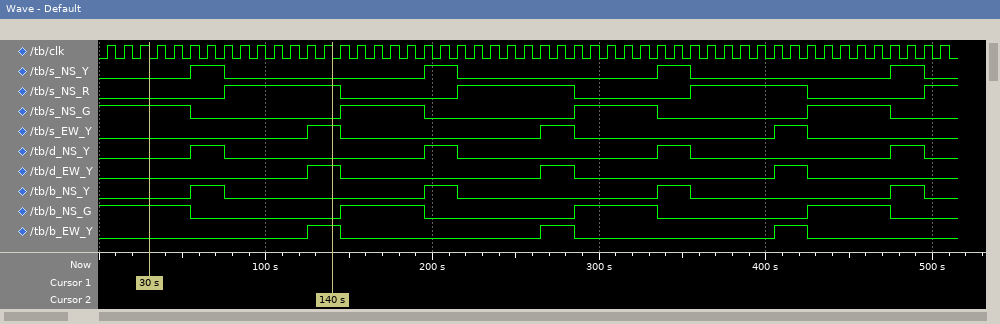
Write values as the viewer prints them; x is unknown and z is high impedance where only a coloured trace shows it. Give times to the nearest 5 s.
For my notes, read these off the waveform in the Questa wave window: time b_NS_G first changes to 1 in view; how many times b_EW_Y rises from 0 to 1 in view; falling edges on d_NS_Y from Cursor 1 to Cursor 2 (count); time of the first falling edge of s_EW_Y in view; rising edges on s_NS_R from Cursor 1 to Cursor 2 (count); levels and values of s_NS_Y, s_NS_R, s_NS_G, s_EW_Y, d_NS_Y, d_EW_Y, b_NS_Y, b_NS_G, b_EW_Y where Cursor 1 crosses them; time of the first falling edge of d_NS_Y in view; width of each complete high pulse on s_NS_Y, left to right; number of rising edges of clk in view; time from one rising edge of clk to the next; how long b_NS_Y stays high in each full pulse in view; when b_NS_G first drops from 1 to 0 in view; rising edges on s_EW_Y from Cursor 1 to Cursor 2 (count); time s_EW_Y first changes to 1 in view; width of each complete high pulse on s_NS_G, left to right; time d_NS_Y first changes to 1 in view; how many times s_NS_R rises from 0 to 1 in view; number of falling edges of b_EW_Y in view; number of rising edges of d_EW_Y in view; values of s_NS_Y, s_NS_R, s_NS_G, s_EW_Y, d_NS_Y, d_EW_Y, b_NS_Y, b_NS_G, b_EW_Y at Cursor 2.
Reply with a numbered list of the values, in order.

1. 145 s
2. 3
3. 1
4. 145 s
5. 1
6. s_NS_Y=0, s_NS_R=0, s_NS_G=1, s_EW_Y=0, d_NS_Y=0, d_EW_Y=0, b_NS_Y=0, b_NS_G=1, b_EW_Y=0
7. 75 s
8. 20 s, 20 s, 20 s, 20 s
9. 51
10. 10 s
11. 20 s, 20 s, 20 s, 20 s
12. 55 s
13. 1
14. 125 s
15. 50 s, 50 s, 50 s
16. 55 s
17. 4
18. 3
19. 3
20. s_NS_Y=0, s_NS_R=1, s_NS_G=0, s_EW_Y=1, d_NS_Y=0, d_EW_Y=1, b_NS_Y=0, b_NS_G=0, b_EW_Y=1
